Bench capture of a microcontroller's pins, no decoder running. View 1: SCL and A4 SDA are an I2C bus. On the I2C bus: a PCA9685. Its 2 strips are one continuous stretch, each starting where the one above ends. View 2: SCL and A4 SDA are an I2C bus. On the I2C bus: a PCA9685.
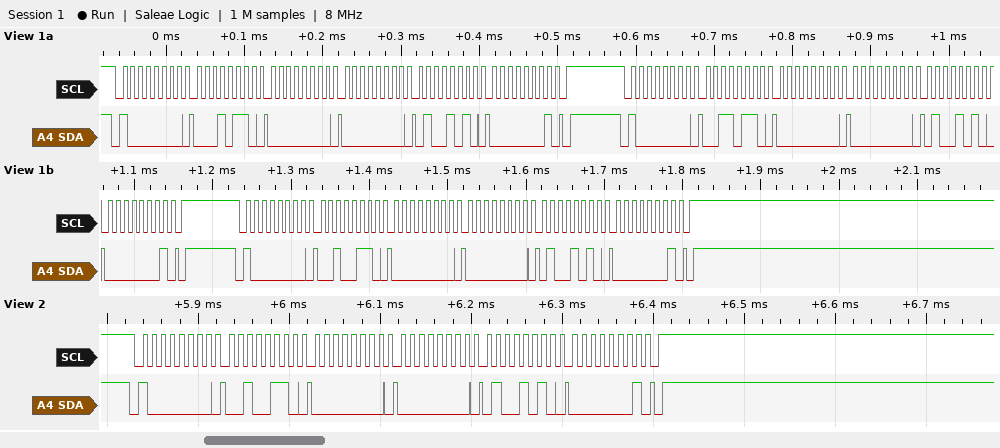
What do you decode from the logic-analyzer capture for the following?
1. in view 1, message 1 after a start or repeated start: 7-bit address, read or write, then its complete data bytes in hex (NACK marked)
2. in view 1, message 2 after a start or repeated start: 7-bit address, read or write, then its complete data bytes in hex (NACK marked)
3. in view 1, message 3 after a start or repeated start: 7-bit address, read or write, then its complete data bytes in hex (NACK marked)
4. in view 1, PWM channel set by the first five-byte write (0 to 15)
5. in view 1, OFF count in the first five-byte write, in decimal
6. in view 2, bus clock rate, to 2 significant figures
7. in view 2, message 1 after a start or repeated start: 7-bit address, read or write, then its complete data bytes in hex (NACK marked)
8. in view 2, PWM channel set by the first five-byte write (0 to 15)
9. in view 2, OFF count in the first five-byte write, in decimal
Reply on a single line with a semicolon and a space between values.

0x40 write: 16 00 00 4A 01; 0x40 write: 36 00 00 4A 01; 0x40 write: 26 00 00 4A 01; 4; 330; 100 kHz; 0x40 write: 26 00 00 4A 01; 8; 330
